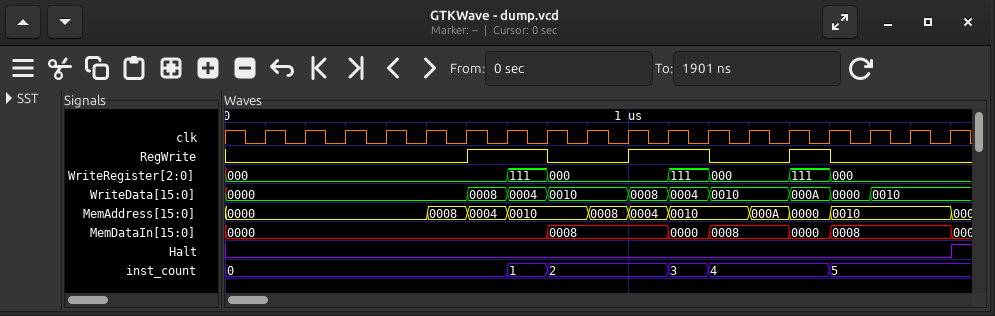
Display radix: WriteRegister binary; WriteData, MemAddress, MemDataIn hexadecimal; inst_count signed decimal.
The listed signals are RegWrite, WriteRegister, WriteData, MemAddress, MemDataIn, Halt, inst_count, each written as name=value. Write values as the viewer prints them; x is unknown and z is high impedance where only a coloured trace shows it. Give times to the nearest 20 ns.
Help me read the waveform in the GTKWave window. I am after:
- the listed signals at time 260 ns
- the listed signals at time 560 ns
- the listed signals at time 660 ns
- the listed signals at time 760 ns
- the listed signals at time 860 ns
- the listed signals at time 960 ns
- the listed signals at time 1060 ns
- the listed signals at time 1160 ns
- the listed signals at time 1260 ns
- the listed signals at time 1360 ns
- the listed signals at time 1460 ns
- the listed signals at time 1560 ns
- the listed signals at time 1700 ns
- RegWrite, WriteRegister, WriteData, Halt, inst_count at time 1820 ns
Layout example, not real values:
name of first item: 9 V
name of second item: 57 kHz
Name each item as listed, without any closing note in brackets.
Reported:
the listed signals at time 260 ns: RegWrite=0, WriteRegister=000, WriteData=0000, MemAddress=0000, MemDataIn=0000, Halt=0, inst_count=0
the listed signals at time 560 ns: RegWrite=0, WriteRegister=000, WriteData=0000, MemAddress=0008, MemDataIn=0000, Halt=0, inst_count=0
the listed signals at time 660 ns: RegWrite=1, WriteRegister=000, WriteData=0008, MemAddress=0004, MemDataIn=0000, Halt=0, inst_count=0
the listed signals at time 760 ns: RegWrite=1, WriteRegister=111, WriteData=0004, MemAddress=0010, MemDataIn=0000, Halt=0, inst_count=1
the listed signals at time 860 ns: RegWrite=0, WriteRegister=000, WriteData=0010, MemAddress=0010, MemDataIn=0008, Halt=0, inst_count=2
the listed signals at time 960 ns: RegWrite=0, WriteRegister=000, WriteData=0010, MemAddress=0008, MemDataIn=0008, Halt=0, inst_count=2
the listed signals at time 1060 ns: RegWrite=1, WriteRegister=000, WriteData=0008, MemAddress=0004, MemDataIn=0008, Halt=0, inst_count=2
the listed signals at time 1160 ns: RegWrite=1, WriteRegister=111, WriteData=0004, MemAddress=0010, MemDataIn=0000, Halt=0, inst_count=3
the listed signals at time 1260 ns: RegWrite=0, WriteRegister=000, WriteData=0010, MemAddress=0010, MemDataIn=0008, Halt=0, inst_count=4
the listed signals at time 1360 ns: RegWrite=0, WriteRegister=000, WriteData=0010, MemAddress=000A, MemDataIn=0008, Halt=0, inst_count=4
the listed signals at time 1460 ns: RegWrite=1, WriteRegister=111, WriteData=000A, MemAddress=0000, MemDataIn=0000, Halt=0, inst_count=4
the listed signals at time 1560 ns: RegWrite=0, WriteRegister=000, WriteData=0000, MemAddress=0010, MemDataIn=0008, Halt=0, inst_count=5
the listed signals at time 1700 ns: RegWrite=0, WriteRegister=000, WriteData=0010, MemAddress=0010, MemDataIn=0008, Halt=0, inst_count=5
RegWrite, WriteRegister, WriteData, Halt, inst_count at time 1820 ns: RegWrite=0, WriteRegister=000, WriteData=0010, Halt=1, inst_count=5
